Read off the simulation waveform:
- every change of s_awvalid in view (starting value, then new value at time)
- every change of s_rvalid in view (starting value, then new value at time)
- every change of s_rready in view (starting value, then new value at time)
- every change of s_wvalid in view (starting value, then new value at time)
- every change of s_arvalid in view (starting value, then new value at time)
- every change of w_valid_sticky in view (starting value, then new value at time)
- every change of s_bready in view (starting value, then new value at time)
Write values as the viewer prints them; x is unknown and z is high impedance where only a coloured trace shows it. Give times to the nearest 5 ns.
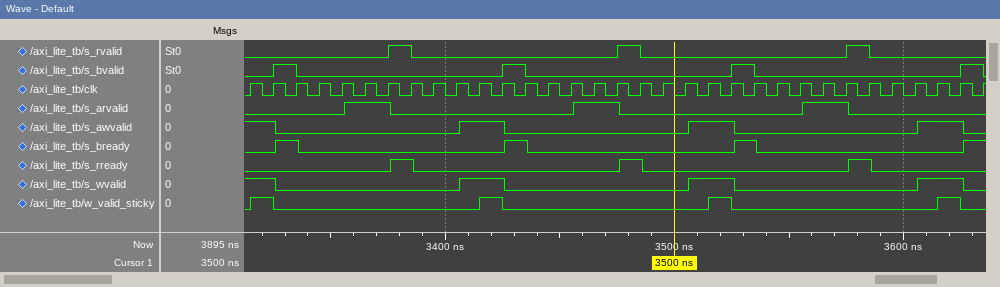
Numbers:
1, 0 at 3325 ns, 1 at 3405 ns, 0 at 3425 ns, 1 at 3505 ns, 0 at 3525 ns, 1 at 3605 ns, 0 at 3625 ns
0, 1 at 3375 ns, 0 at 3385 ns, 1 at 3475 ns, 0 at 3485 ns, 1 at 3575 ns, 0 at 3585 ns
0, 1 at 3375 ns, 0 at 3385 ns, 1 at 3475 ns, 0 at 3485 ns, 1 at 3575 ns, 0 at 3585 ns
1, 0 at 3325 ns, 1 at 3405 ns, 0 at 3425 ns, 1 at 3505 ns, 0 at 3525 ns, 1 at 3605 ns, 0 at 3625 ns
0, 1 at 3355 ns, 0 at 3375 ns, 1 at 3455 ns, 0 at 3475 ns, 1 at 3555 ns, 0 at 3575 ns
0, 1 at 3315 ns, 0 at 3325 ns, 1 at 3415 ns, 0 at 3425 ns, 1 at 3515 ns, 0 at 3525 ns, 1 at 3615 ns, 0 at 3625 ns
0, 1 at 3325 ns, 0 at 3335 ns, 1 at 3425 ns, 0 at 3435 ns, 1 at 3525 ns, 0 at 3535 ns, 1 at 3625 ns
